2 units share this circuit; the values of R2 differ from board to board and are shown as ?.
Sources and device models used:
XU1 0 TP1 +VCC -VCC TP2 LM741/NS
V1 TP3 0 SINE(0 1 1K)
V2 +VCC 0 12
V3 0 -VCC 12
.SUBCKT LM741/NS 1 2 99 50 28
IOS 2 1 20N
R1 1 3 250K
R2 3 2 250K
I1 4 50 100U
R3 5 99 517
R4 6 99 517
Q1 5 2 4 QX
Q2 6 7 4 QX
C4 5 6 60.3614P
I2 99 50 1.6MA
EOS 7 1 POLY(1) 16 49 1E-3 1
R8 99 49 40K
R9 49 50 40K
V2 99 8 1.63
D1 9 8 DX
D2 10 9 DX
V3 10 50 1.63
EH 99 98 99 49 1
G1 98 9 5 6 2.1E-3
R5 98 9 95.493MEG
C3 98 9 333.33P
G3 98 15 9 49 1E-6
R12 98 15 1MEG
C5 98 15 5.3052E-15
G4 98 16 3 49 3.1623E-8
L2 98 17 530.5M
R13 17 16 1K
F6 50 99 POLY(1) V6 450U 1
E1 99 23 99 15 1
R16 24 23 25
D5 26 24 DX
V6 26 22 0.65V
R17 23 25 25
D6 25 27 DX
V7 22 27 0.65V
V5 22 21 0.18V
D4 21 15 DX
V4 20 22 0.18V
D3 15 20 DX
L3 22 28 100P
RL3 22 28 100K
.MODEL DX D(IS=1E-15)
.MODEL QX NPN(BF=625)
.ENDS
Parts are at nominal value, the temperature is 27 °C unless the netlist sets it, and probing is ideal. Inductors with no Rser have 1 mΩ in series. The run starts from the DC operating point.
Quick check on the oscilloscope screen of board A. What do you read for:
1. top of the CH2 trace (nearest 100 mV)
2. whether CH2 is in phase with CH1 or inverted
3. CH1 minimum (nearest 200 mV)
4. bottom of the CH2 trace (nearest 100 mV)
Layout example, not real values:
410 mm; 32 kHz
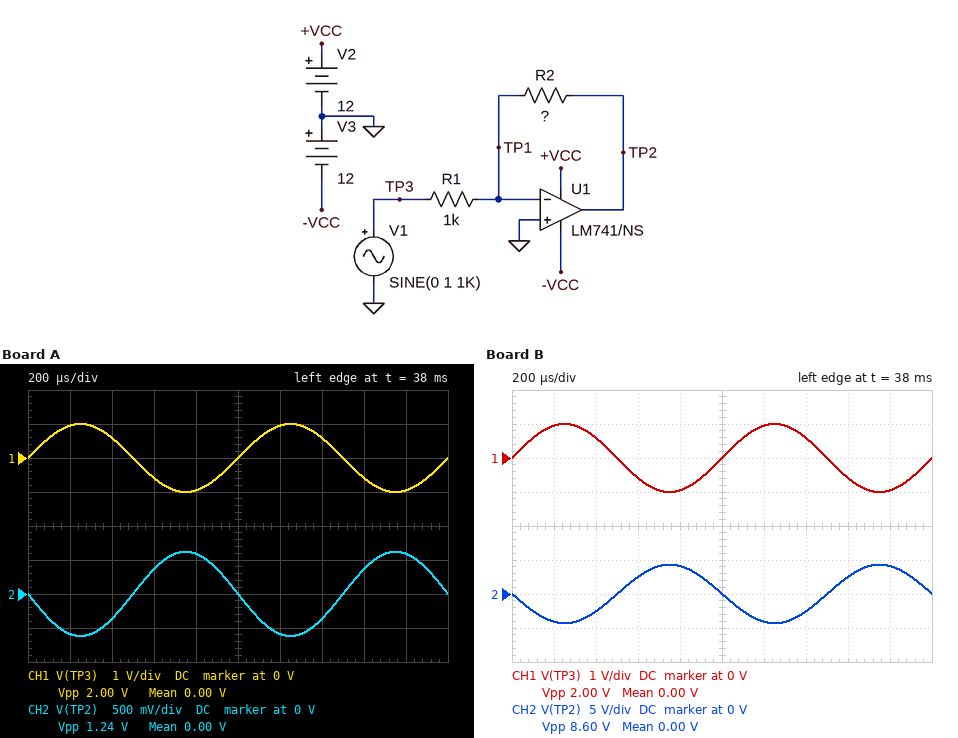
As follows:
600 mV; inverted; -1.0 V; -600 mV
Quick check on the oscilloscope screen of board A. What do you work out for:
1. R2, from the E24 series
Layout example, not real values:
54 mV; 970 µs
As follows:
620 Ω
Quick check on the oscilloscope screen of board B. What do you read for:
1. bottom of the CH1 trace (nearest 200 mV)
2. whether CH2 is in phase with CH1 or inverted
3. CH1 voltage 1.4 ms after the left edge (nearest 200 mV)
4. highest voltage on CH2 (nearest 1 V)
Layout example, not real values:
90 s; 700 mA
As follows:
-1.0 V; inverted; 600 mV; 4 V
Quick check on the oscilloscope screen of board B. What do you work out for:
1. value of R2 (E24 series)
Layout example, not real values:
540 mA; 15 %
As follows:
4.3 kΩ
